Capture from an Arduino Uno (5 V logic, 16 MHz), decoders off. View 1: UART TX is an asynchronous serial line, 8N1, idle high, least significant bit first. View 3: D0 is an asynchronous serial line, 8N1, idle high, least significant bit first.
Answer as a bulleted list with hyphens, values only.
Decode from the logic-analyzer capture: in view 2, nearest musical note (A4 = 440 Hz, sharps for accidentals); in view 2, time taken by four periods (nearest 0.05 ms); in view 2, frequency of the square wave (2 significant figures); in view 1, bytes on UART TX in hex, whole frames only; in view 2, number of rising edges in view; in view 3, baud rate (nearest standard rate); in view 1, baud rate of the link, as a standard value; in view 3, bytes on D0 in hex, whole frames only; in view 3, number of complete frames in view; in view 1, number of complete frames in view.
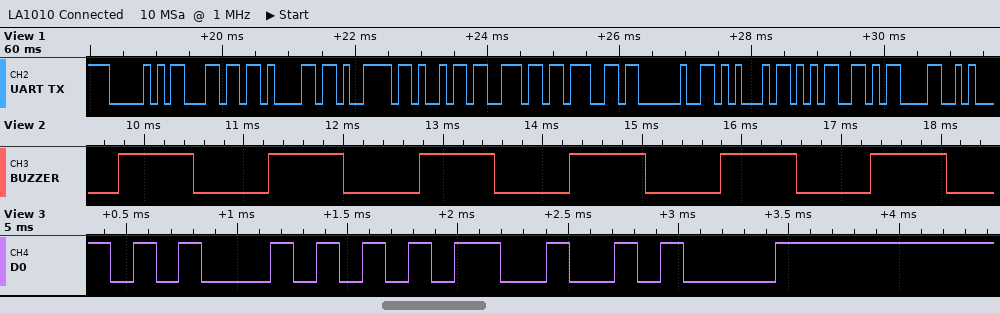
- E5
- 6.05 ms
- 660 Hz
- 0x50 0x6C 0x61 0x79 0x69 0x6E 0x67 0x20 0x45 0x35 0x0D
- 6
- 9600 baud
- 9600 baud
- 0x45 0x35 0x0A
- 3
- 11
